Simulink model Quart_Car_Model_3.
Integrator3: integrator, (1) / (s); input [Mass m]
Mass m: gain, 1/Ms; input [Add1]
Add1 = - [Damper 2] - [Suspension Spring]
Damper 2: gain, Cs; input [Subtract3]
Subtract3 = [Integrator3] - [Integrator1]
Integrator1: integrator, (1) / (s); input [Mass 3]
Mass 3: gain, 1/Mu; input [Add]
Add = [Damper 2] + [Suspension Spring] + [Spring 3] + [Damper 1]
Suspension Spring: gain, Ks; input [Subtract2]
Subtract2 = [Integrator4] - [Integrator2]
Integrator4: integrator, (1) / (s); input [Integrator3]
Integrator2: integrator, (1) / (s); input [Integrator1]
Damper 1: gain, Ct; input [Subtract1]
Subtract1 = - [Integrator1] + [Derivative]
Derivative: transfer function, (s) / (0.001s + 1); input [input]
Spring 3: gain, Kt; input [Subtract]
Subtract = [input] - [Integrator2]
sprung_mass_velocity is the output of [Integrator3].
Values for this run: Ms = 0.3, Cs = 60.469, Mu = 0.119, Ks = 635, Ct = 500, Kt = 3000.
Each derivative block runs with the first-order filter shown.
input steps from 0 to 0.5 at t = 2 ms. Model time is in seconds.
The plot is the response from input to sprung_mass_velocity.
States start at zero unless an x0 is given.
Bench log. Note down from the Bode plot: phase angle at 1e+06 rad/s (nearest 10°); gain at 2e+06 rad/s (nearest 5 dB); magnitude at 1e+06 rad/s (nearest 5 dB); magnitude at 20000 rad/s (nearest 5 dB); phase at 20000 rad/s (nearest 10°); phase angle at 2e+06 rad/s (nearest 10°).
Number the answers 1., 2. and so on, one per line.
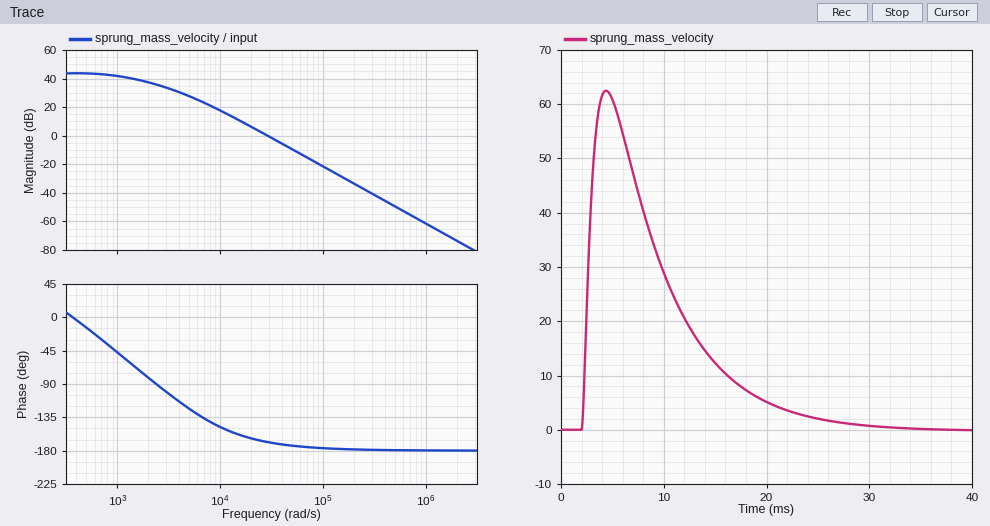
1. -180°
2. -75 dB
3. -60 dB
4. 5 dB
5. -160°
6. -180°
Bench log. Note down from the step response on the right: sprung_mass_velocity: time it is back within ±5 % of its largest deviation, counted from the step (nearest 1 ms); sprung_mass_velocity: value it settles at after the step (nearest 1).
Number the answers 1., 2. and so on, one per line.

1. 21 ms
2. 0
